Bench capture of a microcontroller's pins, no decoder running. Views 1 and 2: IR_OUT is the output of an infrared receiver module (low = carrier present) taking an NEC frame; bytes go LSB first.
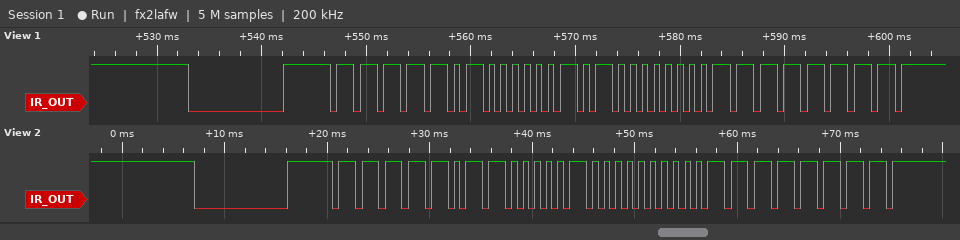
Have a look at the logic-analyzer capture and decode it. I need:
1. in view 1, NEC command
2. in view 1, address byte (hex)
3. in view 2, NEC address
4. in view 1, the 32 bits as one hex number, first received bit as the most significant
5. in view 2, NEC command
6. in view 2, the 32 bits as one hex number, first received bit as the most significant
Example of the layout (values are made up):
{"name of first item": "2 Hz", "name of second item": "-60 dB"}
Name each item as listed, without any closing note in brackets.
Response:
{"in view 1, NEC command": "0x00", "in view 1, address byte": "0x5F", "in view 2, NEC address": "0xDF", "in view 1, the 32 bits as one hex number, first received bit as the most significant": "0xFA0500FF", "in view 2, NEC command": "0x00", "in view 2, the 32 bits as one hex number, first received bit as the most significant": "0xFB0400FF"}
